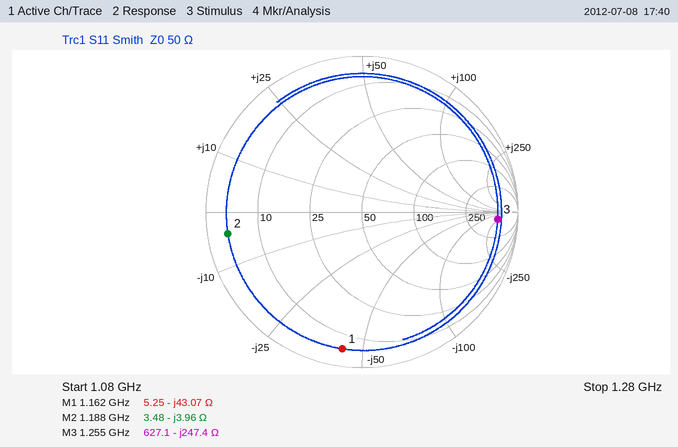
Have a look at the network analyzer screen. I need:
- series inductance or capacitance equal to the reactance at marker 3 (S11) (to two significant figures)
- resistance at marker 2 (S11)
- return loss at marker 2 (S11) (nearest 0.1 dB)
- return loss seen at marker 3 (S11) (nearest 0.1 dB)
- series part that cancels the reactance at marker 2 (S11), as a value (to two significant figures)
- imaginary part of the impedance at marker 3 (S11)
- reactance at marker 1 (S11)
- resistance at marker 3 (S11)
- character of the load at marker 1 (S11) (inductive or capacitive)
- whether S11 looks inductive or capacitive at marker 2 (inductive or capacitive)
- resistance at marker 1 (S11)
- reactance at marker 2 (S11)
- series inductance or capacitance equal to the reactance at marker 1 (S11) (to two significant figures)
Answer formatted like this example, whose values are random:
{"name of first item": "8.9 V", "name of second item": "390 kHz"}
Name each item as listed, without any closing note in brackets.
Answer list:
{"series inductance or capacitance equal to the reactance at marker 3 (S11)": "510 fF", "resistance at marker 2": "3.48 Ω", "return loss at marker 2 (S11)": "1.2 dB", "return loss seen at marker 3 (S11)": "1.2 dB", "series part that cancels the reactance at marker 2 (S11), as a value": "530 pH", "imaginary part of the impedance at marker 3": "-247.4 Ω", "reactance at marker 1": "-43.07 Ω", "resistance at marker 3": "627.1 Ω", "character of the load at marker 1 (S11)": "capacitive", "whether S11 looks inductive or capacitive at marker 2": "capacitive", "resistance at marker 1": "5.25 Ω", "reactance at marker 2": "-3.96 Ω", "series inductance or capacitance equal to the reactance at marker 1 (S11)": "3.2 pF"}
